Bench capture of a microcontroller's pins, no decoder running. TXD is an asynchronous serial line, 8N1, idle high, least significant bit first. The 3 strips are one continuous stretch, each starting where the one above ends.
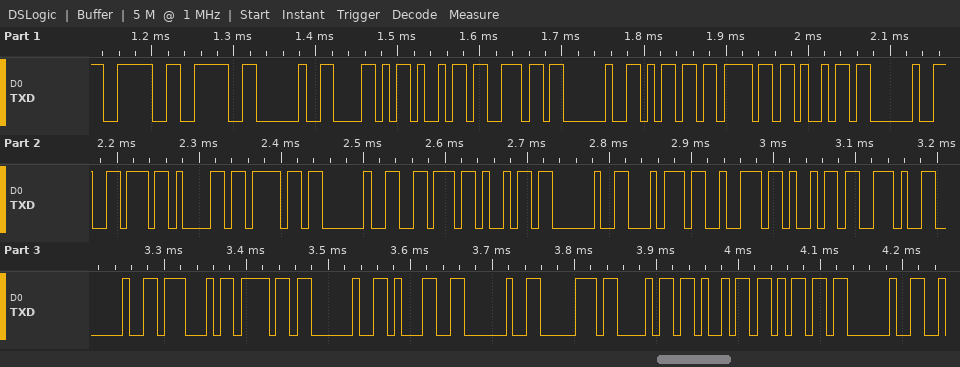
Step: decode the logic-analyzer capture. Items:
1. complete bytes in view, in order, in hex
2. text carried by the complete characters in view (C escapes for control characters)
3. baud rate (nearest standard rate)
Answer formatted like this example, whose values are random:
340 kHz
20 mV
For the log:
3E 3E 20 58 69 6E 20 6D 6F 69 20 76 61 6F 20 76 69 20 74 72 69 2E 20 47 6F 20 31 20 70 68 69 6D 20
">> Xin moi vao vi tri. Go 1 phim "
115200 baud
